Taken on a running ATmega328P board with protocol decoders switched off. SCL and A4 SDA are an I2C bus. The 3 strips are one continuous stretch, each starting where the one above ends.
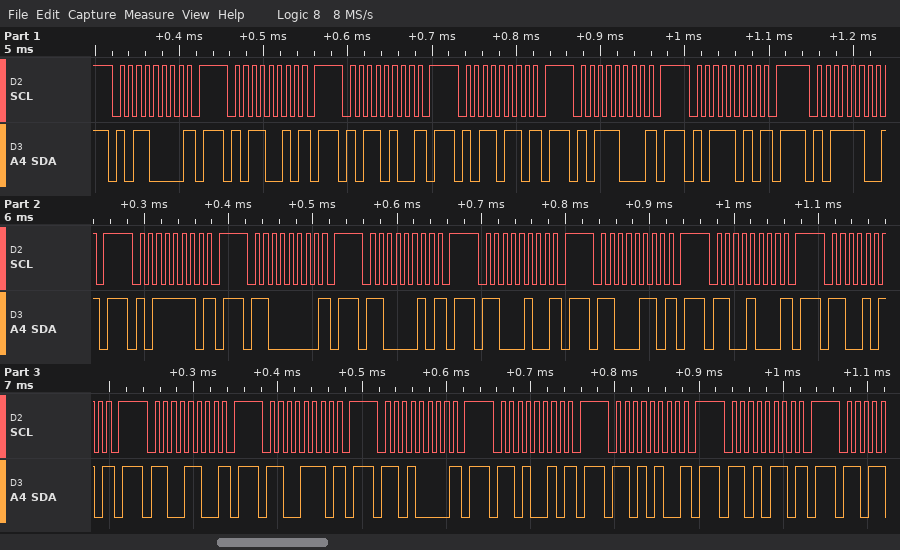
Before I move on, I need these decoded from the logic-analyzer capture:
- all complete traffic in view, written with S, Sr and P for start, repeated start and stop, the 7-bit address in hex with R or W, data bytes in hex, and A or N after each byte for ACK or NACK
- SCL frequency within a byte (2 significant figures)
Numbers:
S 58W N P S 59W N P S 5AW N P S 5BW N P S 5CW N P S 5DW N P S 5EW N P S 5FW N P S 60W N P S 61W N P S 62W N P S 63W N P S 64W N P S 65W N P S 66W N P S 67W N P S 68W N P S 69W N P S 6AW N P S 6BW N P
100 kHz
